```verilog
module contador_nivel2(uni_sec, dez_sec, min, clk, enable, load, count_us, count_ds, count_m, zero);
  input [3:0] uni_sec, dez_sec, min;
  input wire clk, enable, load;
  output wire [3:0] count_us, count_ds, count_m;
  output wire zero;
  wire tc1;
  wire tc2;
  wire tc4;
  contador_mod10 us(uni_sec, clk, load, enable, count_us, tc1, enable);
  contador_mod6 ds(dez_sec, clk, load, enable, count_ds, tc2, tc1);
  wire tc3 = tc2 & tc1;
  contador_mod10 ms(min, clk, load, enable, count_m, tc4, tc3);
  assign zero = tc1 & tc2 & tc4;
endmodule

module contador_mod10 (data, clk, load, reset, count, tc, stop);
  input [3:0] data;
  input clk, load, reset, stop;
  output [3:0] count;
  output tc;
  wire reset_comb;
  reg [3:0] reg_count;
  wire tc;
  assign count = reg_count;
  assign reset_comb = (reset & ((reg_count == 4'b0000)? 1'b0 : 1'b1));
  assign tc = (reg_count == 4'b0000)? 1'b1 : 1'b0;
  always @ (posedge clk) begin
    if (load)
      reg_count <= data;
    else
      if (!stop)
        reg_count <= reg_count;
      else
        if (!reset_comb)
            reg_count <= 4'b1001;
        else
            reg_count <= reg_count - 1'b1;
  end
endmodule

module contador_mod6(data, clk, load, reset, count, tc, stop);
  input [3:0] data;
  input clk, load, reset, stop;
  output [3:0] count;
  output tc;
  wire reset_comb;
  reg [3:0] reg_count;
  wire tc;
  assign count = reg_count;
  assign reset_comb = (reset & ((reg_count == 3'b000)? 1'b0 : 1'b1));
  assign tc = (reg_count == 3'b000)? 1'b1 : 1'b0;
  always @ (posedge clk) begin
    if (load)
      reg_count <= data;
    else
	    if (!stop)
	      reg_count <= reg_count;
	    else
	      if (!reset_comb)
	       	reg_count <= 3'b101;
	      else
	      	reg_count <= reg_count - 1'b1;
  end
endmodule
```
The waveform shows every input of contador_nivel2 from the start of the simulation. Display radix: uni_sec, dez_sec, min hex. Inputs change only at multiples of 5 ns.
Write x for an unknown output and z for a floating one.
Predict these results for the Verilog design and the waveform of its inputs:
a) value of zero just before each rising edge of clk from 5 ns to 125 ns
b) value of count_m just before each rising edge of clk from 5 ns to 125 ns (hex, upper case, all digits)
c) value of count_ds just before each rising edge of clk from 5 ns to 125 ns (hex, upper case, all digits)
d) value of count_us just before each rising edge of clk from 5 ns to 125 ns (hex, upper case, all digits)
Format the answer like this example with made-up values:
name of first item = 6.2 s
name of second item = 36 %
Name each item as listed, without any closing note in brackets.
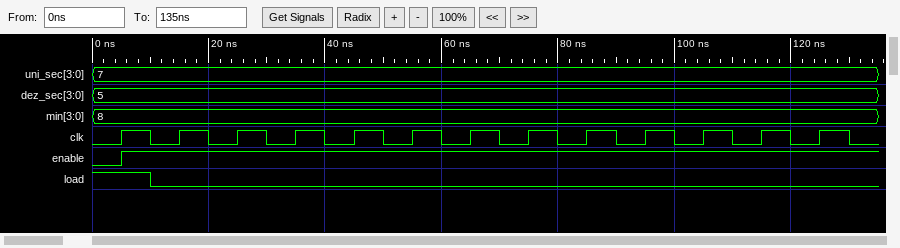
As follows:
value of zero just before each rising edge of clk from 5 ns to 125 ns = x 0 0 0 0 0 0 0 0 0 0 0 0
value of count_m just before each rising edge of clk from 5 ns to 125 ns = x, 8, 8, 8, 8, 8, 8, 8, 8, 8, 8, 8, 8
value of count_ds just before each rising edge of clk from 5 ns to 125 ns = x, 5, 5, 5, 5, 5, 5, 5, 5, 4, 4, 4, 4
value of count_us just before each rising edge of clk from 5 ns to 125 ns = x, 7, 6, 5, 4, 3, 2, 1, 0, 9, 8, 7, 6
